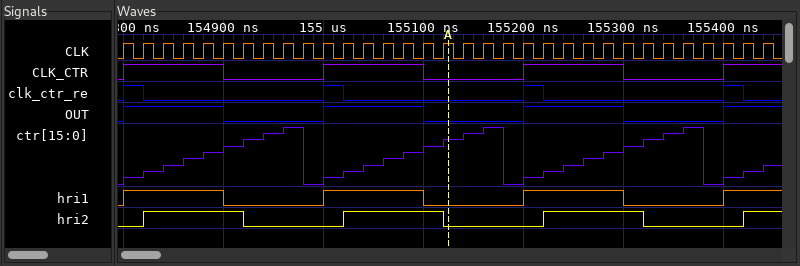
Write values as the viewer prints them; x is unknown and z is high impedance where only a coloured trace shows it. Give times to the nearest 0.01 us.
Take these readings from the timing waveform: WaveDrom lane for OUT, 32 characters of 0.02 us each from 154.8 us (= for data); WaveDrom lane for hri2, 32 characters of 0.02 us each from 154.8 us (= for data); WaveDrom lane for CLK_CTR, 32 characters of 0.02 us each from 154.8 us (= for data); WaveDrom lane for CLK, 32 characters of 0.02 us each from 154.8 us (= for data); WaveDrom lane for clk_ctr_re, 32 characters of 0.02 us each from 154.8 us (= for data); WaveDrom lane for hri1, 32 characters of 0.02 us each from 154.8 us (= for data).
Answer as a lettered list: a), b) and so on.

a) {name: 'OUT', wave: '1....0....1....0....1....0....1.'}
b) {name: 'hri2', wave: '01....0....1....0....1....0....1'}
c) {name: 'CLK_CTR', wave: '1....0....1....0....1....0....1.'}
d) {name: 'CLK', wave: 'p...............................'}
e) {name: 'clk_ctr_re', wave: '10........10........10........10'}
f) {name: 'hri1', wave: '1....0....1....0....1....0....1.'}
